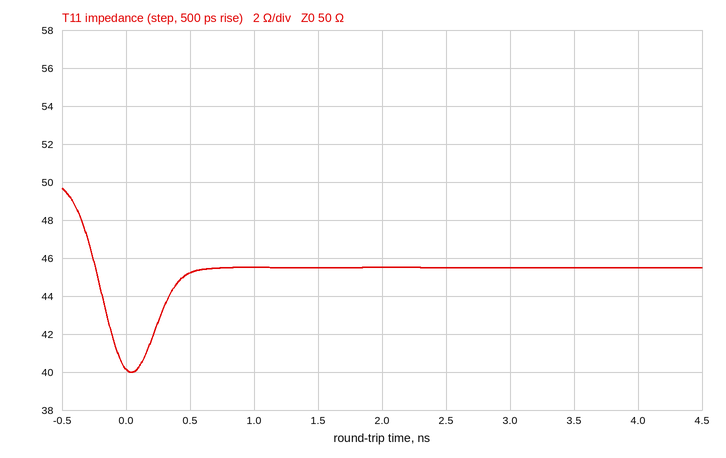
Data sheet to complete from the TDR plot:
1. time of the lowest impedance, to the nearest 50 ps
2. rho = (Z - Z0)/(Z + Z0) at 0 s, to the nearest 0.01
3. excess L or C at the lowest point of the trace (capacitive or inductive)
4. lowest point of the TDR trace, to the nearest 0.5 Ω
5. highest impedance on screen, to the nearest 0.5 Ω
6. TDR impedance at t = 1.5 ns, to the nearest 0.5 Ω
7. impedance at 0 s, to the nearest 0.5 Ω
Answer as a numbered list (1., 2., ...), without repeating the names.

1. 50 ps
2. -0.11
3. capacitive
4. 40.0 Ω
5. 49.5 Ω
6. 45.5 Ω
7. 40.0 Ω
